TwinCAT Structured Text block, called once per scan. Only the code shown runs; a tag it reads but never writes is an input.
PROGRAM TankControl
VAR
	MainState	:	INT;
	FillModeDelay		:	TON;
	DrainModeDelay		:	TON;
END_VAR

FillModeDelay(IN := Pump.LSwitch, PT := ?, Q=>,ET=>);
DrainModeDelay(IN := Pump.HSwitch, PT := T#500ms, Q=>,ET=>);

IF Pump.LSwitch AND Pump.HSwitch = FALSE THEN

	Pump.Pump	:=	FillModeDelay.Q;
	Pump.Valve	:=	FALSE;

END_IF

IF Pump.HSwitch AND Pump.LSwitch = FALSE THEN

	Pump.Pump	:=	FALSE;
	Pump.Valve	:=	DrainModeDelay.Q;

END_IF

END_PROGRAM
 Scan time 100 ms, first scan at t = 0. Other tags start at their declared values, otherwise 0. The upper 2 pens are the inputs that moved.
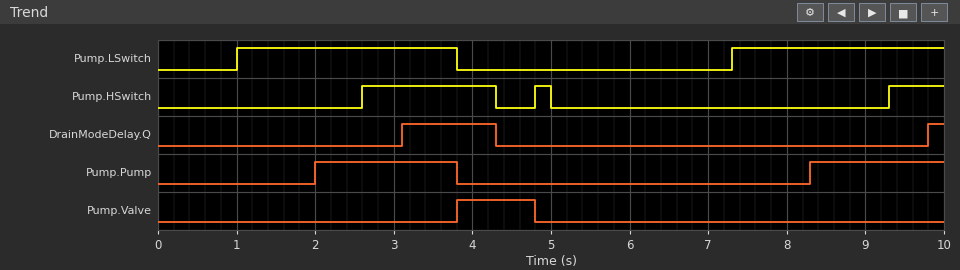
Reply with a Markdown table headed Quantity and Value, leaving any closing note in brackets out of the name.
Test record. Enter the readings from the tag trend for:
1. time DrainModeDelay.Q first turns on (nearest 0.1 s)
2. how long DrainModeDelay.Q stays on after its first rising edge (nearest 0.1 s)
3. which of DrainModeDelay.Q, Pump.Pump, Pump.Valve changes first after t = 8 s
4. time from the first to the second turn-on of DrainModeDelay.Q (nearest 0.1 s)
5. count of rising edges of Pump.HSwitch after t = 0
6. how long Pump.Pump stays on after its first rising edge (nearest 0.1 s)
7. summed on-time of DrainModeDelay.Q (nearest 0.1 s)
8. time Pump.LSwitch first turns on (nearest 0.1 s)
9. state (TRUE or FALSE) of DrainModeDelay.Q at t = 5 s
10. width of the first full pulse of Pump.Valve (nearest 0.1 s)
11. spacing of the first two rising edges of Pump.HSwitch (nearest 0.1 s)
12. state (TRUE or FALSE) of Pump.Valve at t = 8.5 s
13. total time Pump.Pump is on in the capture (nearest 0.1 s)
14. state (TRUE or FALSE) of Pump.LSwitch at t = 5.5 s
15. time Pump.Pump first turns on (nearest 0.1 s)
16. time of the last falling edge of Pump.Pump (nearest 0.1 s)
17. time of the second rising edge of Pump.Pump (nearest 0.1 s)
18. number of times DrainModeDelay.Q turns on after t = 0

| Quantity | Value |
|---|---|
| time DrainModeDelay.Q first turns on | 3.1 s |
| how long DrainModeDelay.Q stays on after its first rising edge | 1.2 s |
| which of DrainModeDelay.Q, Pump.Pump, Pump.Valve changes first after t = 8 s | Pump.Pump |
| time from the first to the second turn-on of DrainModeDelay.Q | 6.7 s |
| count of rising edges of Pump.HSwitch after t = 0 | 3 |
| how long Pump.Pump stays on after its first rising edge | 1.8 s |
| summed on-time of DrainModeDelay.Q | 1.4 s |
| time Pump.LSwitch first turns on | 1.0 s |
| state (TRUE or FALSE) of DrainModeDelay.Q at t = 5 s | FALSE |
| width of the first full pulse of Pump.Valve | 1.0 s |
| spacing of the first two rising edges of Pump.HSwitch | 2.2 s |
| state (TRUE or FALSE) of Pump.Valve at t = 8.5 s | FALSE |
| total time Pump.Pump is on in the capture | 3.5 s |
| state (TRUE or FALSE) of Pump.LSwitch at t = 5.5 s | FALSE |
| time Pump.Pump first turns on | 2.0 s |
| time of the last falling edge of Pump.Pump | 3.8 s |
| time of the second rising edge of Pump.Pump | 8.3 s |
| number of times DrainModeDelay.Q turns on after t = 0 | 2 |
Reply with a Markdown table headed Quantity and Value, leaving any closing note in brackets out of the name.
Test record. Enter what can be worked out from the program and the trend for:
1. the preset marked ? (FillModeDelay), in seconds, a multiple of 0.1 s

| Quantity | Value |
|---|---|
| the preset marked ? (FillModeDelay), in seconds, a multiple of 0.1 s | 1.0 s |
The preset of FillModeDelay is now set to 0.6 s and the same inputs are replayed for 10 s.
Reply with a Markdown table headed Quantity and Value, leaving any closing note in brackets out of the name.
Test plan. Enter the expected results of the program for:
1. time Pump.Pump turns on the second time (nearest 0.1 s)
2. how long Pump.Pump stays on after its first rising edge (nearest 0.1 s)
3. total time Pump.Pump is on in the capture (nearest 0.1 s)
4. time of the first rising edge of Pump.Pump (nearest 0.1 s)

| Quantity | Value |
|---|---|
| time Pump.Pump turns on the second time | 7.9 s |
| how long Pump.Pump stays on after its first rising edge | 2.2 s |
| total time Pump.Pump is on in the capture | 4.3 s |
| time of the first rising edge of Pump.Pump | 1.6 s |
